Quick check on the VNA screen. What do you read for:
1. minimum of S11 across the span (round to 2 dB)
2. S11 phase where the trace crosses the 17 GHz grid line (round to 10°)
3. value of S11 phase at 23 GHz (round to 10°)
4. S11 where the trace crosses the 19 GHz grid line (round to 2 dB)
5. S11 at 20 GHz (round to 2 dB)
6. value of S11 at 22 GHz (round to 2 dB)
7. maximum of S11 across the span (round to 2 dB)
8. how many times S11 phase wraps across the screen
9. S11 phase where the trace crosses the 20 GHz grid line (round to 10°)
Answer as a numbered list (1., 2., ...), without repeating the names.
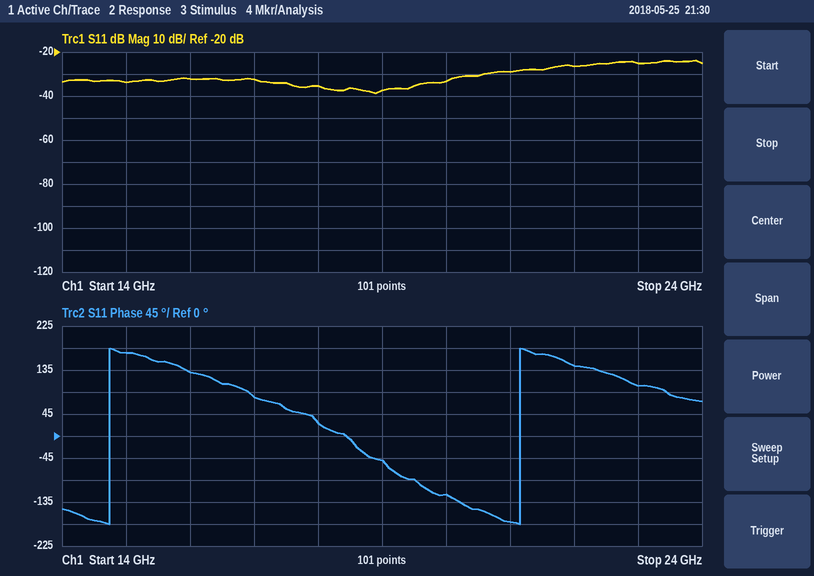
1. -38 dB
2. 80°
3. 100°
4. -38 dB
5. -34 dB
6. -26 dB
7. -24 dB
8. 2
9. -120°
